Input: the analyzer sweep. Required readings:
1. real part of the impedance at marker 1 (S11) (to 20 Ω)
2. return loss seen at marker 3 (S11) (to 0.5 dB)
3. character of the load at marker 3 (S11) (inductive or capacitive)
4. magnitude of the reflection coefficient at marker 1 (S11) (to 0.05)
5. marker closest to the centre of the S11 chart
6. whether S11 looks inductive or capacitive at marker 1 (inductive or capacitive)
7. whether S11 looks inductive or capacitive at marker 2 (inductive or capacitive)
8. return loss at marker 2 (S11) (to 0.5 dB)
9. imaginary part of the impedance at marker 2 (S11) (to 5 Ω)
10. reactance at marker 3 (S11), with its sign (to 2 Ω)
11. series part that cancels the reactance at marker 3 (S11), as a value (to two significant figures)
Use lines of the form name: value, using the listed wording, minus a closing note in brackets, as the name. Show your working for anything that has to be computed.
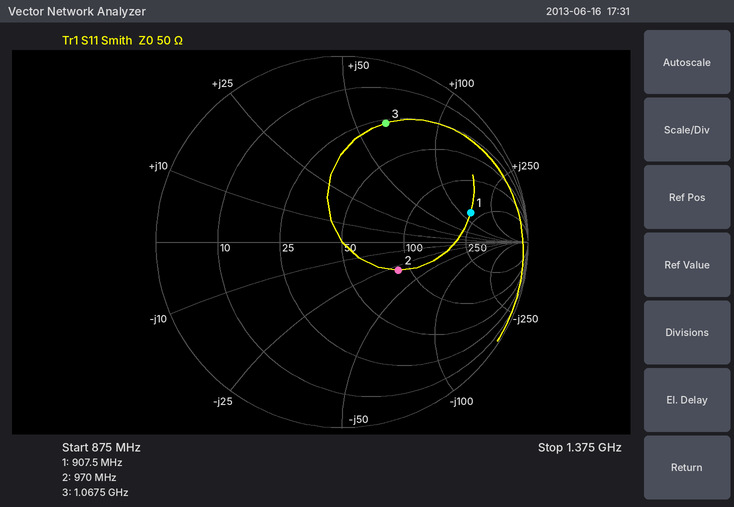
real part of the impedance at marker 1 (S11): 200 Ω
return loss seen at marker 3 (S11): 3.5 dB
character of the load at marker 3 (S11): inductive
magnitude of the reflection coefficient at marker 1 (S11): 0.70
marker closest to the centre of the S11 chart: marker 2
whether S11 looks inductive or capacitive at marker 1: inductive
whether S11 looks inductive or capacitive at marker 2: capacitive
return loss at marker 2 (S11): 9.5 dB
imaginary part of the impedance at marker 2 (S11): -30 Ω
reactance at marker 3 (S11), with its sign: +64 Ω
series part that cancels the reactance at marker 3 (S11), as a value: C = 1/(2π × 1.0675 GHz × 64 Ω) ≈ 2.3 pF
